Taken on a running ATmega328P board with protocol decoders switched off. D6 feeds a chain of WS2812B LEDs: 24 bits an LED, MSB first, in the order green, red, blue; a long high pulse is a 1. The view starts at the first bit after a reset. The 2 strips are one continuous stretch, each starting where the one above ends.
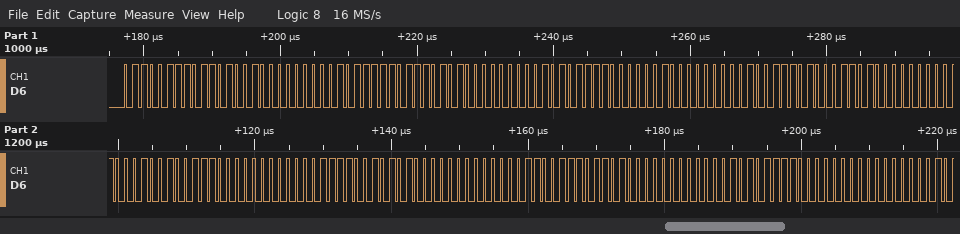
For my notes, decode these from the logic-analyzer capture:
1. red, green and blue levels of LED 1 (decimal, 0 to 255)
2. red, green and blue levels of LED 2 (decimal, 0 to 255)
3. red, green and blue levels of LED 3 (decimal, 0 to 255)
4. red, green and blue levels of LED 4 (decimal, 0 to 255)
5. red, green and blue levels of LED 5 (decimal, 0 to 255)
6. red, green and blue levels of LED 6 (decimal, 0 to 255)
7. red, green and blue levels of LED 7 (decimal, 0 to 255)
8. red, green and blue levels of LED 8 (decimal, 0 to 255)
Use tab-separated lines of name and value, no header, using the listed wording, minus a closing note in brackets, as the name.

red, green and blue levels of LED 1	105, 103, 0
red, green and blue levels of LED 2	117, 95, 0
red, green and blue levels of LED 3	129, 87, 0
red, green and blue levels of LED 4	141, 78, 0
red, green and blue levels of LED 5	156, 68, 0
red, green and blue levels of LED 6	168, 60, 0
red, green and blue levels of LED 7	180, 51, 0
red, green and blue levels of LED 8	192, 43, 0
